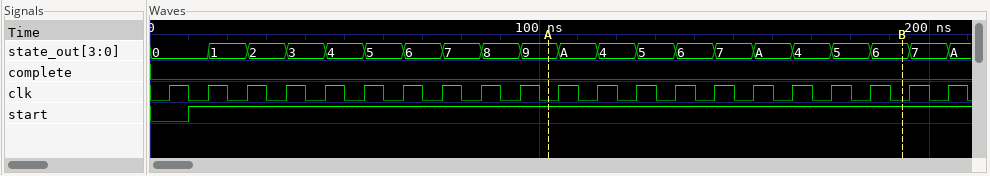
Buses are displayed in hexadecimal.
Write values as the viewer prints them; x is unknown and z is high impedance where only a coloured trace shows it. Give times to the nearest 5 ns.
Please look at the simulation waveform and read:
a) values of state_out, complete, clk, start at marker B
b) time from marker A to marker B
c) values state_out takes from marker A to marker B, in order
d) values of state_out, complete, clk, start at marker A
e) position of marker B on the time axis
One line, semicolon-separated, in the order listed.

state_out=6, complete=0, clk=0, start=1; 90 ns; 9, A, 4, 5, 6, 7, A, 4, 5, 6; state_out=9, complete=0, clk=0, start=1; 195 ns
